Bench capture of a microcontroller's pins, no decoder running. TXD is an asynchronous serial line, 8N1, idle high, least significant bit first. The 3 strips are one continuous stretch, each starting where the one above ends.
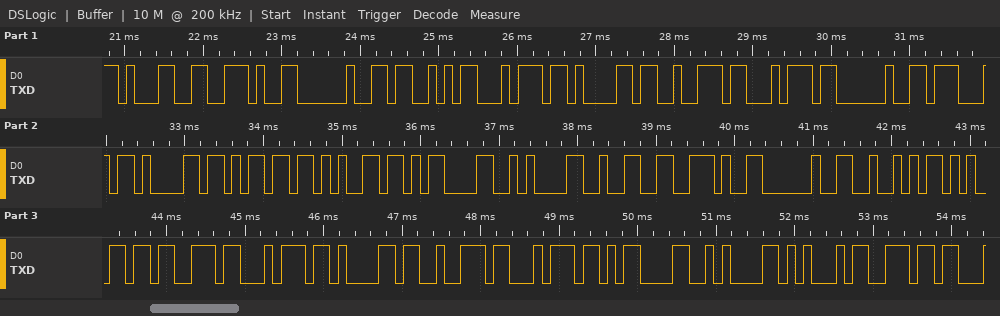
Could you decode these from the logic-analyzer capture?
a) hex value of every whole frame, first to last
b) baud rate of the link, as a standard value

0x31 0x2E 0x20 0x53 0x74 0x61 0x72 0x74 0x20 0x47 0x61 0x6D 0x65 0x0D 0x0A 0x32 0x2E 0x20 0x52 0x65 0x73 0x74 0x61 0x72 0x74 0x0D 0x0A 0x45 0x6E
9600 baud
